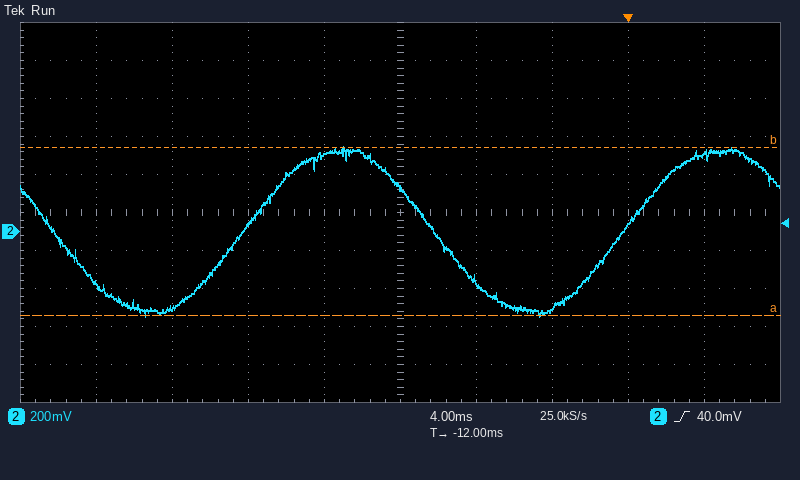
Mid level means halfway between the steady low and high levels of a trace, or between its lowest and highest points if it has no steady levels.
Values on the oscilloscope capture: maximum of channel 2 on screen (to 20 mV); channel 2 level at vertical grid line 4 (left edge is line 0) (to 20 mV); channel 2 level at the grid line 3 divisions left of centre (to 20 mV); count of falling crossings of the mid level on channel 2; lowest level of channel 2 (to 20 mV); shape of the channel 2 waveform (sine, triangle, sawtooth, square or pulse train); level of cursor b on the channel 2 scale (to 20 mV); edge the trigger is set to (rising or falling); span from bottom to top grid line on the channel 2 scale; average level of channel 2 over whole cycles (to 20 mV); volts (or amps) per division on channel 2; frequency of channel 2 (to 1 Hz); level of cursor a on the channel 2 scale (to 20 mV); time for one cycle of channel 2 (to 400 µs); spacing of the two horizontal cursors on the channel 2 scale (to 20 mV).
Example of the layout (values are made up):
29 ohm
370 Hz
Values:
440 mV
400 mV
-400 mV
2
-440 mV
sine
440 mV
rising
2 V
0 mV
200 mV
50 Hz
-440 mV
20.0 ms
880 mV
